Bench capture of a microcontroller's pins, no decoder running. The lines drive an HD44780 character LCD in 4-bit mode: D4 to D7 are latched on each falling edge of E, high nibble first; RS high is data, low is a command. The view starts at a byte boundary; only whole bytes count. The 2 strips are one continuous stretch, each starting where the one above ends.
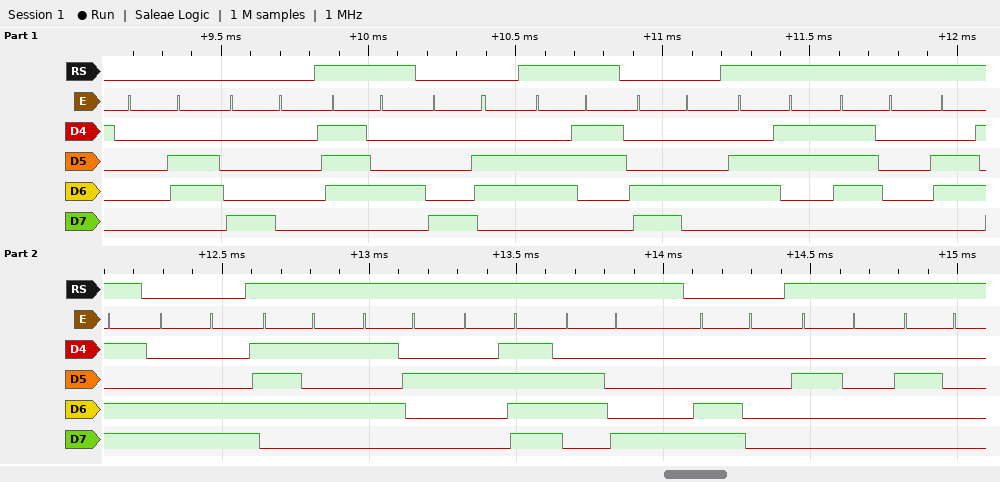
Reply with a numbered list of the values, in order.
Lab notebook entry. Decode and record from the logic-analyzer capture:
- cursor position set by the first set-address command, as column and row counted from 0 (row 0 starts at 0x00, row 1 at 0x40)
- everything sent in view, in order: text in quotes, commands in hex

1. column 0, row 0
2. 0x06 0x80 "t" 0x86 "c" 0xC4 "cpm" 0xCC "uR/h" 0xC0 "  "
